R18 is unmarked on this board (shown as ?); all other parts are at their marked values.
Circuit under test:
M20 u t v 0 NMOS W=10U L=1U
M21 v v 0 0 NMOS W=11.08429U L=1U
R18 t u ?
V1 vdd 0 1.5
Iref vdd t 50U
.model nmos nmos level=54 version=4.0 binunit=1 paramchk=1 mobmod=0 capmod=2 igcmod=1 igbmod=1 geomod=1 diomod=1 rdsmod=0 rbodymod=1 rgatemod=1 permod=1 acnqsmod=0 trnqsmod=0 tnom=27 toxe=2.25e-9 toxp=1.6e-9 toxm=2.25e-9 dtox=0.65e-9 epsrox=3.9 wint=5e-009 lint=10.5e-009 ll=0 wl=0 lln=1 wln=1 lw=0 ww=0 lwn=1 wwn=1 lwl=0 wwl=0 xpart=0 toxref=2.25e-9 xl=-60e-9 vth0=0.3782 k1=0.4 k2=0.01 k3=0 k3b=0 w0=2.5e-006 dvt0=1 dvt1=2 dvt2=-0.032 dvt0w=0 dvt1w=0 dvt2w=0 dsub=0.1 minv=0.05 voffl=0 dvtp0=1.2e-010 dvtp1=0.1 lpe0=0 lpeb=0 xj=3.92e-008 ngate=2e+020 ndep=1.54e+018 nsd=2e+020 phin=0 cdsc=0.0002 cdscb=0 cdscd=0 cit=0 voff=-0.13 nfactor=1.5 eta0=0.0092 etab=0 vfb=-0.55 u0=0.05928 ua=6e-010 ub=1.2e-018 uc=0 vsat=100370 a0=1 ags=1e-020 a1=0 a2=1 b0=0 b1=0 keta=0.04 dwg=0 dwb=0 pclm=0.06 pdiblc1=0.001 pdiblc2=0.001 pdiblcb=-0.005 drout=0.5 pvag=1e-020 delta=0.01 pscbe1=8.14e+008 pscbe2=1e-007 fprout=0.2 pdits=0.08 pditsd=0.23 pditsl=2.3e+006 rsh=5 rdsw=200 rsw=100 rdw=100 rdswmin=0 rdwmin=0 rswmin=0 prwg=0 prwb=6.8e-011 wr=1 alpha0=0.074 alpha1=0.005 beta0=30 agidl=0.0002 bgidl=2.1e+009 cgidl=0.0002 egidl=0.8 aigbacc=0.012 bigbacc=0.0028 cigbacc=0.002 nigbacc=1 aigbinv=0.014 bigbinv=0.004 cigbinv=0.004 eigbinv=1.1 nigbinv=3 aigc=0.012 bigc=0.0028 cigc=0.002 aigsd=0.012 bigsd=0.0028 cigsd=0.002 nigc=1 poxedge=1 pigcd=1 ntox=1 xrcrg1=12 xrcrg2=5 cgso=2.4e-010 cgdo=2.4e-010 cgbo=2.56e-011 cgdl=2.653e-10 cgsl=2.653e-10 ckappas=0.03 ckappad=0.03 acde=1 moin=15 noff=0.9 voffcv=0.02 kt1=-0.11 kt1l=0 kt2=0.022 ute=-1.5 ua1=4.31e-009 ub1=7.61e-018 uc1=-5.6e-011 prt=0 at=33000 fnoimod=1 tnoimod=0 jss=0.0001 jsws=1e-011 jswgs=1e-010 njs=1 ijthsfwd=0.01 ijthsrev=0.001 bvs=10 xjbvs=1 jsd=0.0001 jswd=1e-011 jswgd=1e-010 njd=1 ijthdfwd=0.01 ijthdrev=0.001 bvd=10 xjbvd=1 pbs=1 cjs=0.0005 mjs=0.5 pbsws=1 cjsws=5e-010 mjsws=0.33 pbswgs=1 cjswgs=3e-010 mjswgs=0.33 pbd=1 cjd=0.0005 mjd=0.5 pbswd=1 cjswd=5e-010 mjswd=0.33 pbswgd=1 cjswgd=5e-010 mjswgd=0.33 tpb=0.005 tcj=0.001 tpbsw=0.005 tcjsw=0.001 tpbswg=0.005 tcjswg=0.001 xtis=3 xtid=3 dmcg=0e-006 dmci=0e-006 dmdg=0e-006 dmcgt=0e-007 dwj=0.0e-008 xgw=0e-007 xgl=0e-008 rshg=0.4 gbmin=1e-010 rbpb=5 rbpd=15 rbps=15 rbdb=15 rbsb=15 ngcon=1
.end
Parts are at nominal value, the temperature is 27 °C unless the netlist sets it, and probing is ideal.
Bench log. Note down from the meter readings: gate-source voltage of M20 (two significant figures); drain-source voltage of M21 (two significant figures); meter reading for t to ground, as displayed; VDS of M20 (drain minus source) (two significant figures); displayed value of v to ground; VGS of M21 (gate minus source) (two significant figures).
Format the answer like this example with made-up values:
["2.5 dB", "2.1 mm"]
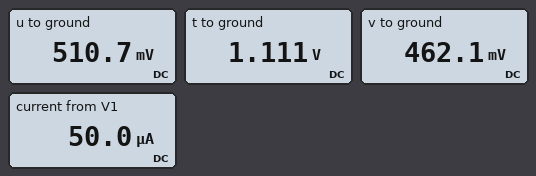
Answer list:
["650 mV", "460 mV", "1.111 V", "49 mV", "462.1 mV", "460 mV"]
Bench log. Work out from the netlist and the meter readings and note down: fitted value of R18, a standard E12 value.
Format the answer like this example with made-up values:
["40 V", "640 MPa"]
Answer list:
["12 kΩ"]
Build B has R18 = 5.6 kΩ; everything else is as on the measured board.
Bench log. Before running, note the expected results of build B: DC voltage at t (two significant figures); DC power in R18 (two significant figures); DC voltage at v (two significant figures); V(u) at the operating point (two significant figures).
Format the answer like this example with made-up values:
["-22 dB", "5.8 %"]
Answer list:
["1.0 V", "14 µW", "460 mV", "750 mV"]
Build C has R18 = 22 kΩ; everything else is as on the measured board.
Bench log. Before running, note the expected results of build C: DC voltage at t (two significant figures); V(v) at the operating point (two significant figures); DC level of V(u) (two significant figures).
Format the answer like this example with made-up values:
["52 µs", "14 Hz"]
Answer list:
["1.6 V", "460 mV", "480 mV"]
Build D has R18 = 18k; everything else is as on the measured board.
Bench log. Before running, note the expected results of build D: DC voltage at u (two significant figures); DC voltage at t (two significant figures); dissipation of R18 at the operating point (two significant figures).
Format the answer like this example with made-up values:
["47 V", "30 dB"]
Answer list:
["480 mV", "1.4 V", "45 µW"]
